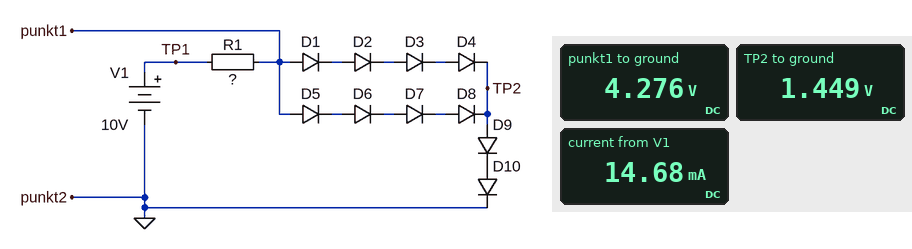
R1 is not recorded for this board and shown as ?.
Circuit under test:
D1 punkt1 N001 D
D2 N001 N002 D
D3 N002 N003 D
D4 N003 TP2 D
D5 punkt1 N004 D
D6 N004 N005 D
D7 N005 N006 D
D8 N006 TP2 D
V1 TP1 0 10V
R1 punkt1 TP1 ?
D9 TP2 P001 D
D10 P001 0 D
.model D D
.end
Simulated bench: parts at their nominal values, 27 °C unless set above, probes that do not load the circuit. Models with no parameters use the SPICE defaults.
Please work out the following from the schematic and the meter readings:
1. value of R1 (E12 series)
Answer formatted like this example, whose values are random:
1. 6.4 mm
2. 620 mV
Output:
1. 390 Ω
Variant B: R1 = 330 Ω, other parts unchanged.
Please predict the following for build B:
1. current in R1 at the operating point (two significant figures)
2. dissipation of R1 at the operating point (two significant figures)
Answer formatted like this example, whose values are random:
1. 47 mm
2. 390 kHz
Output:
1. 17 mA
2. 98 mW
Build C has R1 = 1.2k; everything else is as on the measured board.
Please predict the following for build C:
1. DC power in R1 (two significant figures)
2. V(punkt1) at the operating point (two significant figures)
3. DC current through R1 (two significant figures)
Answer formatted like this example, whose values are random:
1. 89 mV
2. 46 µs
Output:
1. 29 mW
2. 4.1 V
3. 4.9 mA
